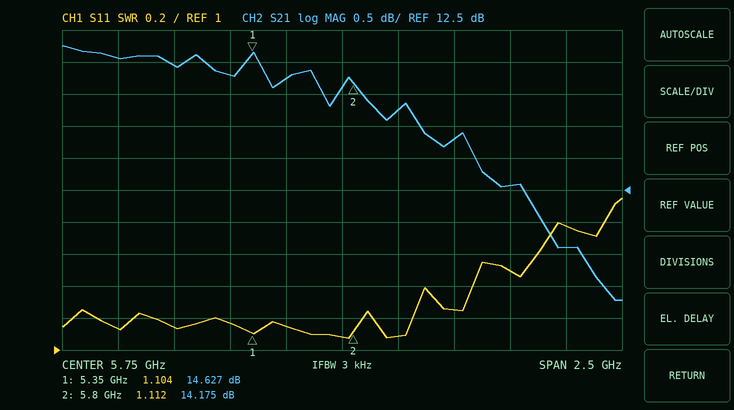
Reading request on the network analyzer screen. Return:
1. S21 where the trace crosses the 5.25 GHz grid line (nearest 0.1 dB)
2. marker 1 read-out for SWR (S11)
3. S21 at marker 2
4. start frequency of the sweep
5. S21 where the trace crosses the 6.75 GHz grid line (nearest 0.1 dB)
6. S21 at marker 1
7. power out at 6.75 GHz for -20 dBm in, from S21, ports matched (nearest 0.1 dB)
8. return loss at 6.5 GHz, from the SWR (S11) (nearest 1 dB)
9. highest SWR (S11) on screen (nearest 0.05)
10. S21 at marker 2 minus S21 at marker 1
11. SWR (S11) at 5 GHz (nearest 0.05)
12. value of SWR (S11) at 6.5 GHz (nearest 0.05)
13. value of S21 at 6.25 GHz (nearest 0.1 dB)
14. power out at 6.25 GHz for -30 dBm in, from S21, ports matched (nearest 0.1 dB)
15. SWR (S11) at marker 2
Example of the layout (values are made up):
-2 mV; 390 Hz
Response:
14.3 dB; 1.104; 14.175 dB; 4.5 GHz; 11.6 dB; 14.627 dB; -8.4 dBm; 14 dB; 1.95; -0.452 dB; 1.15; 1.50; 13.3 dB; -16.7 dBm; 1.112
